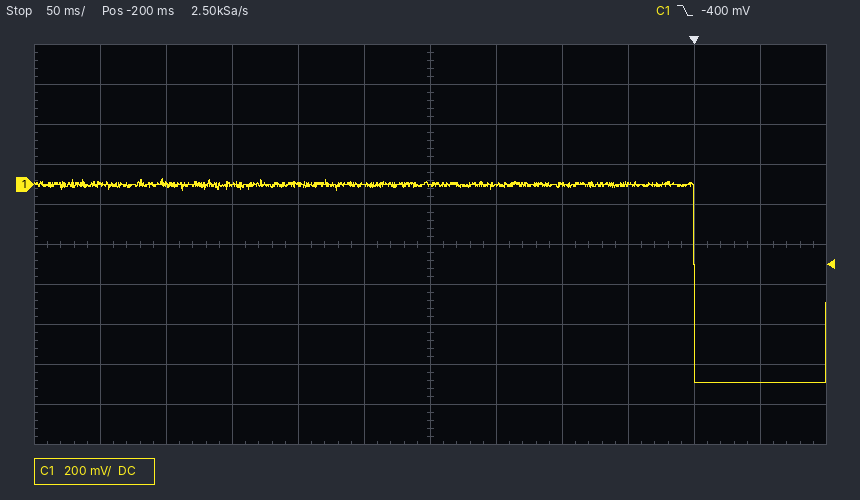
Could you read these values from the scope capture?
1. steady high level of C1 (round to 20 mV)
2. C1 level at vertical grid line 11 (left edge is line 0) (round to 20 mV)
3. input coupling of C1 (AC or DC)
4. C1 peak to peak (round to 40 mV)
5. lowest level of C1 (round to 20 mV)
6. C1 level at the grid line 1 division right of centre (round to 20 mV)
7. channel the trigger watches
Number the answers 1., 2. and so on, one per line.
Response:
1. 0 mV
2. -1.00 V
3. DC
4. 1.04 V
5. -1.00 V
6. 0 mV
7. C1
